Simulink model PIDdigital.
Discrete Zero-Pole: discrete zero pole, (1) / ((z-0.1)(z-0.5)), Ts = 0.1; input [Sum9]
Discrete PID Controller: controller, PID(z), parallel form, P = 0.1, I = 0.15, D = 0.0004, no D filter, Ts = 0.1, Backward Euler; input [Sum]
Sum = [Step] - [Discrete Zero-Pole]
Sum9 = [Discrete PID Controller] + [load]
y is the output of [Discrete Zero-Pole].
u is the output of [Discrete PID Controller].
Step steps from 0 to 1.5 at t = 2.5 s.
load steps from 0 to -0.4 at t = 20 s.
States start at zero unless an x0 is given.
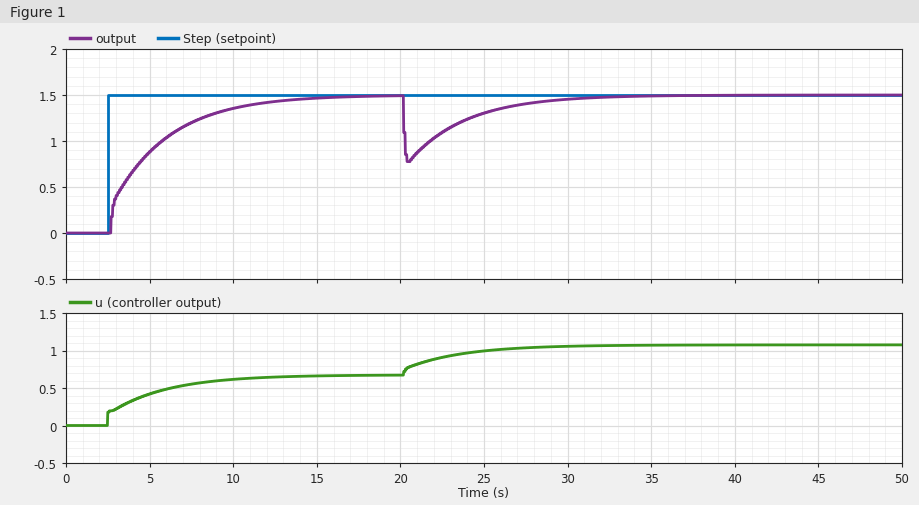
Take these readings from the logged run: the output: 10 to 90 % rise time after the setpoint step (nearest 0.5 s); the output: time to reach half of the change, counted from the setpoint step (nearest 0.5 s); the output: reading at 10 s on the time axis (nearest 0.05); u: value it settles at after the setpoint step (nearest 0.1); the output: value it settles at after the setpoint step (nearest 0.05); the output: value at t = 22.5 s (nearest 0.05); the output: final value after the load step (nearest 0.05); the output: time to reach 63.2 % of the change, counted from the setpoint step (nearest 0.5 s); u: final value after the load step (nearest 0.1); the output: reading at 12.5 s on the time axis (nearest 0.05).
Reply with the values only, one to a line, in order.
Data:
7.0 s
2.0 s
1.35
0.7
1.50
1.10
1.50
3.0 s
1.1
1.45
